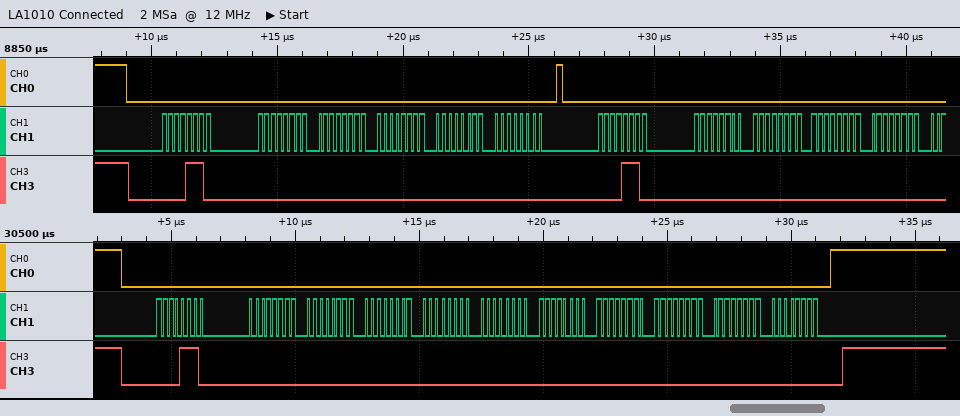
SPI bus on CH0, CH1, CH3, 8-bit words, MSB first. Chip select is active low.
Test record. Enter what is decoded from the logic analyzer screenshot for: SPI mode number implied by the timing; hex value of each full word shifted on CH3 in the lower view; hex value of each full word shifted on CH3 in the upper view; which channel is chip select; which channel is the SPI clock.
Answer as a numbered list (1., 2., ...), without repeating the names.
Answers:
1. 0
2. 0E, 00, 00, 00, 00, 00, 00, 00, 00, 00, 00
3. 0E, 00, 00, 00, 00, 00, 0E, 00, 00, 00, 00
4. CH0
5. CH1
